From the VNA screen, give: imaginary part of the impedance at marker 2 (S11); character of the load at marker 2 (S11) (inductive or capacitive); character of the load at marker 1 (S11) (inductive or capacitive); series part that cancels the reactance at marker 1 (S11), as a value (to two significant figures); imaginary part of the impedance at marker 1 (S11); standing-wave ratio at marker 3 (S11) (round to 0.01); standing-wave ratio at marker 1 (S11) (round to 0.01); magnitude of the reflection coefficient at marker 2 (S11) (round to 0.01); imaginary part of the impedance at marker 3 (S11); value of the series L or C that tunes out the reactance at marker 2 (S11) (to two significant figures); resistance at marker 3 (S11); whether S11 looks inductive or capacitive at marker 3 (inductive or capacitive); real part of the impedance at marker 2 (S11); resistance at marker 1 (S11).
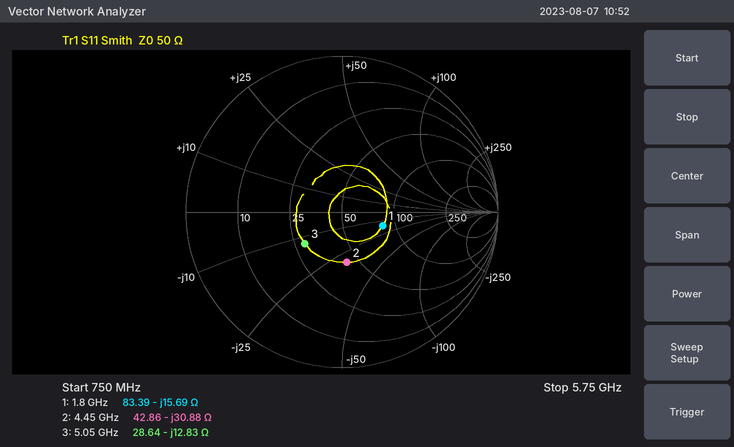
-30.88 Ω
capacitive
capacitive
1.4 nH
-15.69 Ω
1.91
1.76
0.32
-12.83 Ω
1.1 nH
28.64 Ω
capacitive
42.86 Ω
83.39 Ω
